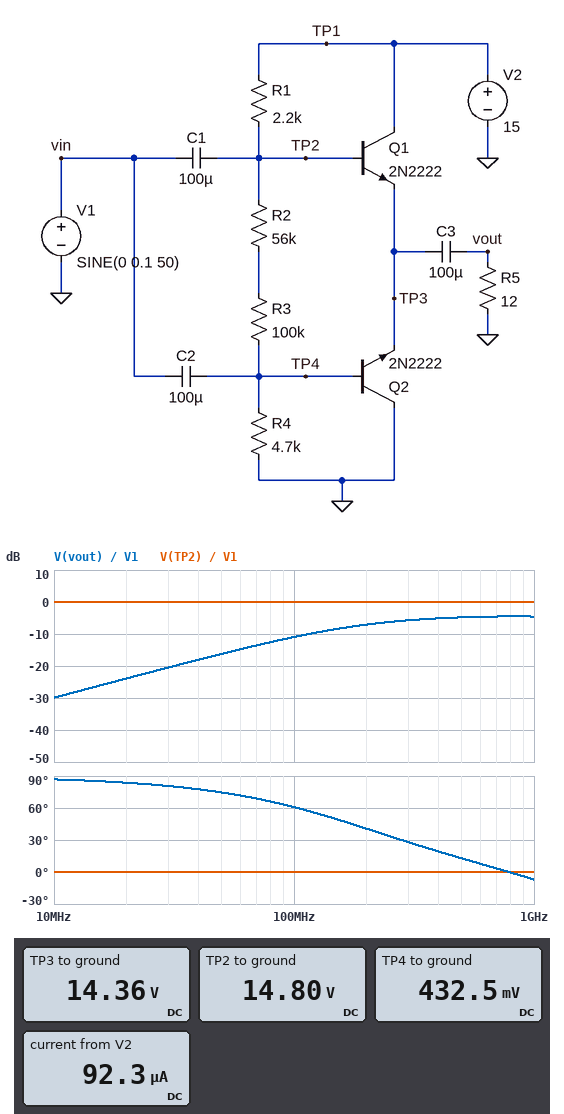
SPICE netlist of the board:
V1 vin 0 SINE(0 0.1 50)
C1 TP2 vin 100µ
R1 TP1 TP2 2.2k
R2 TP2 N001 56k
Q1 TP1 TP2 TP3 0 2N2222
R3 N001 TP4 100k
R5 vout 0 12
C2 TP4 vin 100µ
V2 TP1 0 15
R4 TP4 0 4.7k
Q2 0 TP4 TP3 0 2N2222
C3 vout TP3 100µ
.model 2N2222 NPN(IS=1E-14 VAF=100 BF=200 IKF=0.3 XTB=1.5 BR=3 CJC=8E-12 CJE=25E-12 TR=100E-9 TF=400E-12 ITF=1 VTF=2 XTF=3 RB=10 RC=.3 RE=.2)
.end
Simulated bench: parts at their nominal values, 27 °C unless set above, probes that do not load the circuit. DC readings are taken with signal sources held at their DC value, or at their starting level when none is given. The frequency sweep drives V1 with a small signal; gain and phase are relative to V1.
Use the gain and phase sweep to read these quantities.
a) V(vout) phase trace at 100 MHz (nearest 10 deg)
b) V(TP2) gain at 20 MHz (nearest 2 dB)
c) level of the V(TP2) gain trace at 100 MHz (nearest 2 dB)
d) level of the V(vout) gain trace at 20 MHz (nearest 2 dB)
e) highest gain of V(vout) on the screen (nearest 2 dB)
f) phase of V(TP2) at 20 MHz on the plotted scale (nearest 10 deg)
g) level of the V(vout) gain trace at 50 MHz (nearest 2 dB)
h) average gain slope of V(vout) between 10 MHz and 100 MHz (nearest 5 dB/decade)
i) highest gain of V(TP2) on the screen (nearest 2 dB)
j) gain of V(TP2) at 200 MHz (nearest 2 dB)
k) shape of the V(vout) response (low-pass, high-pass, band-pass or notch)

60 deg
0 dB
0 dB
-24 dB
-4 dB
0 deg
-16 dB
20 dB/decade
0 dB
0 dB
high-pass
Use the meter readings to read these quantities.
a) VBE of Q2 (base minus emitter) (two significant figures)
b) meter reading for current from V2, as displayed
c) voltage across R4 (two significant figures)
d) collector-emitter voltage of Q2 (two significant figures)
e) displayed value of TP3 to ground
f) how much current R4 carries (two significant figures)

-14 V
92.3 µA
430 mV
-14 V
14.36 V
92 µA
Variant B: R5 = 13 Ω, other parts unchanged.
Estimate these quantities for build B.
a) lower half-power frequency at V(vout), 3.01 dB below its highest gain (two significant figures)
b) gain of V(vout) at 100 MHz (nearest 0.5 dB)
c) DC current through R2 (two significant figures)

170 MHz
-10.5 dB
92 µA
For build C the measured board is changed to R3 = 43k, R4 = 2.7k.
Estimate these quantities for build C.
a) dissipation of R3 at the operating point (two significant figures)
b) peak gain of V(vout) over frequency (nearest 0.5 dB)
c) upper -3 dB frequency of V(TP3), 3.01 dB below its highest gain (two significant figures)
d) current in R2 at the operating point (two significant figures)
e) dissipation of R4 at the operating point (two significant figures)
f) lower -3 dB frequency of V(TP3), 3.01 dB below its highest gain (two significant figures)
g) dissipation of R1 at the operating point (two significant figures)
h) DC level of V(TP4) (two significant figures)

900 µW
-4.5 dB
3.3 GHz
140 µA
56 µW
190 MHz
46 µW
390 mV
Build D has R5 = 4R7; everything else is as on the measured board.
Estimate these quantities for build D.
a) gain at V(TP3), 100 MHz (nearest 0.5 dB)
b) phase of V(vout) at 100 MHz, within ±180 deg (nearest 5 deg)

-18.5 dB
70 deg
